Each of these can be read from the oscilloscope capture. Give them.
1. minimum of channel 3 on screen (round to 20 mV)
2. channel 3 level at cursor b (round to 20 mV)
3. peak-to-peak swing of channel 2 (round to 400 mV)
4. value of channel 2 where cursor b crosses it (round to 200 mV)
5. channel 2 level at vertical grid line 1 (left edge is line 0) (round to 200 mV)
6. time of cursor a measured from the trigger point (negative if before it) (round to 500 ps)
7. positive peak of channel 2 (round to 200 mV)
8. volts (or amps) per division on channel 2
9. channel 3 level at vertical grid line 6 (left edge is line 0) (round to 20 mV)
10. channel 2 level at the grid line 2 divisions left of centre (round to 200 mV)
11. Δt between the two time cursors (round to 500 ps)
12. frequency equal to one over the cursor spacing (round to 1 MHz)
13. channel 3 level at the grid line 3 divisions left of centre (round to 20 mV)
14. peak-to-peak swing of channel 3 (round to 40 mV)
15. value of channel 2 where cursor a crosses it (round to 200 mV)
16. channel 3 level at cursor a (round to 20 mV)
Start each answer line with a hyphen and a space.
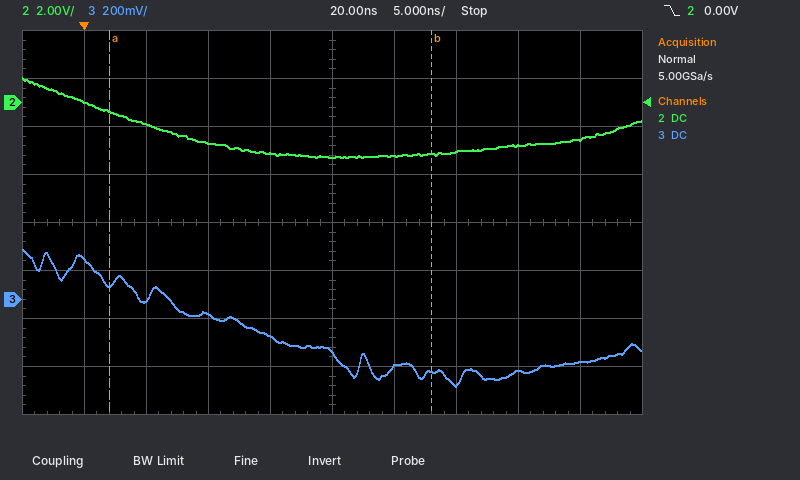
- -360 mV
- -300 mV
- 3.2 V
- -2.2 V
- 0.0 V
- +2.0 ns
- 1.0 V
- 2 V
- -280 mV
- -1.6 V
- 26.0 ns
- 38 MHz
- 0 mV
- 560 mV
- -400 mV
- 60 mV
